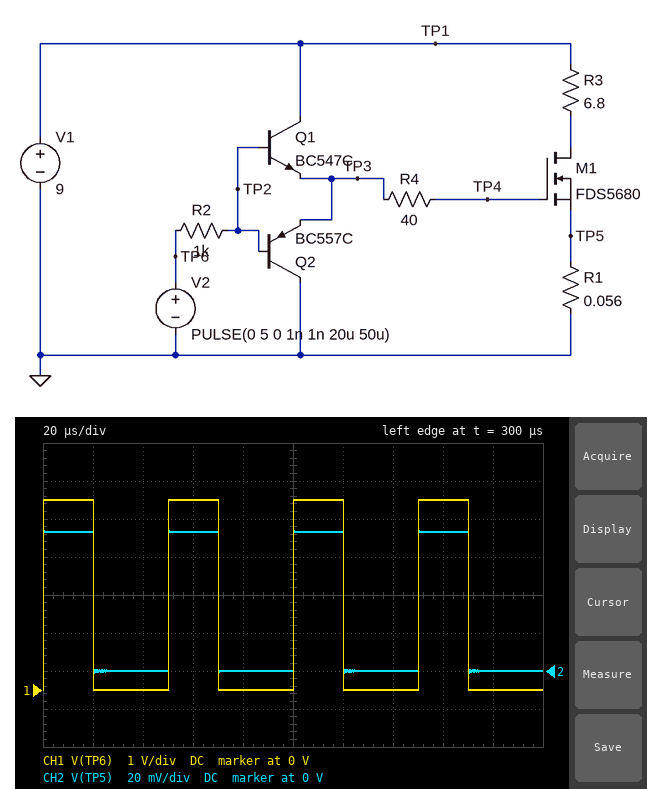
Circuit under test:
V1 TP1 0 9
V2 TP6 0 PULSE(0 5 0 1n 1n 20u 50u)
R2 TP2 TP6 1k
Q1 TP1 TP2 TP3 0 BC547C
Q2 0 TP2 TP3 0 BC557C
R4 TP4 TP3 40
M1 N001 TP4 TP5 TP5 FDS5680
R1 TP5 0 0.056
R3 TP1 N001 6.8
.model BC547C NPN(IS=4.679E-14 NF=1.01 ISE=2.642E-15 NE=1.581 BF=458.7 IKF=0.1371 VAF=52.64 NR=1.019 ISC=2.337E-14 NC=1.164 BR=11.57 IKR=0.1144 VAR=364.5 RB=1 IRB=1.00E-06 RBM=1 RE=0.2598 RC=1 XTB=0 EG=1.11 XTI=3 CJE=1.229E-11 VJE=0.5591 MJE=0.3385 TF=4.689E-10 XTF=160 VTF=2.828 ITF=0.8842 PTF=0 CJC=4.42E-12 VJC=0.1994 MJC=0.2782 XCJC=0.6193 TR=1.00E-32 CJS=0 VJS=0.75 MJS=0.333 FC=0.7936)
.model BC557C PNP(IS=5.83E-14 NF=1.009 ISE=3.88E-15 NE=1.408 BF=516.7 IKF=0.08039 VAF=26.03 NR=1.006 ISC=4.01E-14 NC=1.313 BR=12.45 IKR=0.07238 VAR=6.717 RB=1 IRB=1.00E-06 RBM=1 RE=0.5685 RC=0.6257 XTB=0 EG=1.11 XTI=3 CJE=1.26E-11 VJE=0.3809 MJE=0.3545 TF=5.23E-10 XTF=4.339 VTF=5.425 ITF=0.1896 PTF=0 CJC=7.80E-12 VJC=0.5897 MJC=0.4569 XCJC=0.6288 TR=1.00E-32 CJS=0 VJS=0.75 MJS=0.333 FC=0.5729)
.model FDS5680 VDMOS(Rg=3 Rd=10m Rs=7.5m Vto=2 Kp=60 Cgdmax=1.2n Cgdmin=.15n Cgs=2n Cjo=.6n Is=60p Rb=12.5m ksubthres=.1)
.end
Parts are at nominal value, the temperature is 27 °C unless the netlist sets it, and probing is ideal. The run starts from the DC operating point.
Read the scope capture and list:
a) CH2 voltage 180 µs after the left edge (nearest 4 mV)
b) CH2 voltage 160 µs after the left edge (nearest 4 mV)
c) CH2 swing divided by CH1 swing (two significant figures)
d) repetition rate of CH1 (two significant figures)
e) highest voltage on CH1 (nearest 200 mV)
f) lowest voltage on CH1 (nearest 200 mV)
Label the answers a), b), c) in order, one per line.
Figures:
a) 0 V
b) 72 mV
c) 0.015
d) 20 kHz
e) 5.0 V
f) 0 V
